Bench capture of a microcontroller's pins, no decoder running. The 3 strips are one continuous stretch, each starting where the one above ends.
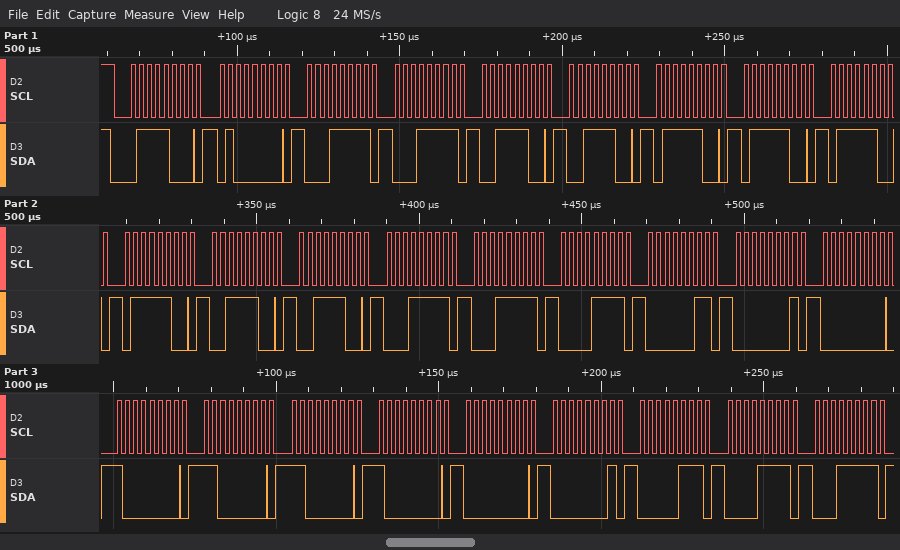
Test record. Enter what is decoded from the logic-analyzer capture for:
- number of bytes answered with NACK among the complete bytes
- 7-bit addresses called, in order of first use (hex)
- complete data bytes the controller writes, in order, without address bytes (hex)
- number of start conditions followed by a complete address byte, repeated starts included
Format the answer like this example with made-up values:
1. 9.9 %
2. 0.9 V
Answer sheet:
1. 0
2. 0x3C
3. 40 1F 1F 3C 3C 7C 7C 7C 7C 3C 3C 1F 1F 0F 03 01 00 80 C0 C0 80 00 01 07 0F 1F
4. 1
